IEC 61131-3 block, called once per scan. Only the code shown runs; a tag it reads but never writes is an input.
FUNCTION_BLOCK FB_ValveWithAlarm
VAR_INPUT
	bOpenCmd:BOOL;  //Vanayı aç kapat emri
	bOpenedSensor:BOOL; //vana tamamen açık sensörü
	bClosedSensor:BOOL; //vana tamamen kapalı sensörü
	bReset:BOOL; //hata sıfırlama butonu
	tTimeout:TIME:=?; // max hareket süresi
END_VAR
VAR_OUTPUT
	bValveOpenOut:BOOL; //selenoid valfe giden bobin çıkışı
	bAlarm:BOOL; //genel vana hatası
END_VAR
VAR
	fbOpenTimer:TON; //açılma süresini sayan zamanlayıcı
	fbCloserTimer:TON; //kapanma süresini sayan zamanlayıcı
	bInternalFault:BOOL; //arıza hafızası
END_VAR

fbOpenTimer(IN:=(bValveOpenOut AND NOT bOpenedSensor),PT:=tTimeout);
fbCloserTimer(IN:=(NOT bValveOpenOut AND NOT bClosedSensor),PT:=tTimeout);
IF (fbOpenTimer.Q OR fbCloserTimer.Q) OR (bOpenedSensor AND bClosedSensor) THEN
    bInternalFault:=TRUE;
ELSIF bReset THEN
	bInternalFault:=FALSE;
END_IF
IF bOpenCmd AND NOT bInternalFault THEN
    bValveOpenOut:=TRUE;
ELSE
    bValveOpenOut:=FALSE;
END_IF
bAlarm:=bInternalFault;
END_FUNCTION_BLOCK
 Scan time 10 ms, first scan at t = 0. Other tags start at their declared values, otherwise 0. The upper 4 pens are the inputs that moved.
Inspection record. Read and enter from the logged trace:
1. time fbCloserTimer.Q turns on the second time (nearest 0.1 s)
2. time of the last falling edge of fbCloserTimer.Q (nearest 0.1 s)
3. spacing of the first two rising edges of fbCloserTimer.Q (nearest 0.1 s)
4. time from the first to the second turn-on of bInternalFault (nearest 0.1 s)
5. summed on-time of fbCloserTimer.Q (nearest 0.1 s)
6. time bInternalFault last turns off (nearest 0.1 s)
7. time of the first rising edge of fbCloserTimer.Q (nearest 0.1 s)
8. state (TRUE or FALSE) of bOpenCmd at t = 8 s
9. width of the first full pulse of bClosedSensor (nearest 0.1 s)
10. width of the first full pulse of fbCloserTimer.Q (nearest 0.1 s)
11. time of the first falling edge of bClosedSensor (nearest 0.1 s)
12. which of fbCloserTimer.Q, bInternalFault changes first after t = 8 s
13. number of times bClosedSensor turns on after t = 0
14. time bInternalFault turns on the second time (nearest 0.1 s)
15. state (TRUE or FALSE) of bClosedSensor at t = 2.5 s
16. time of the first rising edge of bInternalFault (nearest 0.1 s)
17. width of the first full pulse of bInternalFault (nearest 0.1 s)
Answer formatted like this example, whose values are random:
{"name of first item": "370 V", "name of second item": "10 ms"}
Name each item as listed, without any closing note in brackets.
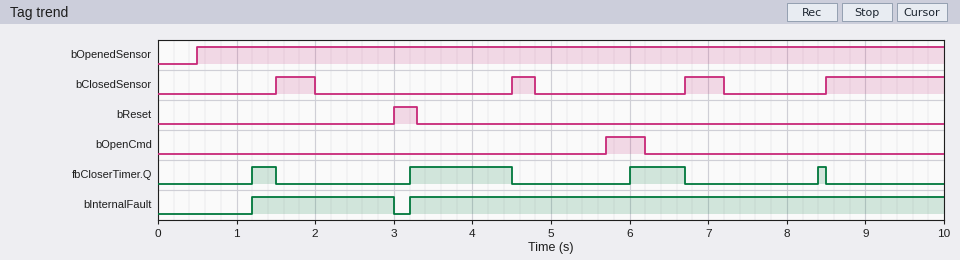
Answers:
{"time fbCloserTimer.Q turns on the second time": "3.2 s", "time of the last falling edge of fbCloserTimer.Q": "8.5 s", "spacing of the first two rising edges of fbCloserTimer.Q": "2.0 s", "time from the first to the second turn-on of bInternalFault": "2.0 s", "summed on-time of fbCloserTimer.Q": "2.4 s", "time bInternalFault last turns off": "3.0 s", "time of the first rising edge of fbCloserTimer.Q": "1.2 s", "state (TRUE or FALSE) of bOpenCmd at t = 8 s": "FALSE", "width of the first full pulse of bClosedSensor": "0.5 s", "width of the first full pulse of fbCloserTimer.Q": "0.3 s", "time of the first falling edge of bClosedSensor": "2.0 s", "which of fbCloserTimer.Q, bInternalFault changes first after t = 8 s": "fbCloserTimer.Q", "number of times bClosedSensor turns on after t = 0": "4", "time bInternalFault turns on the second time": "3.2 s", "state (TRUE or FALSE) of bClosedSensor at t = 2.5 s": "FALSE", "time of the first rising edge of bInternalFault": "1.2 s", "width of the first full pulse of bInternalFault": "1.8 s"}
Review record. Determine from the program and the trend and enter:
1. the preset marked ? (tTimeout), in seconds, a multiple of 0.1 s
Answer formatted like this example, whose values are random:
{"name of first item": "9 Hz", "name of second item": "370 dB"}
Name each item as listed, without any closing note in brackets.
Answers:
{"the preset marked ? (tTimeout), in seconds, a multiple of 0.1 s": "1.2 s"}
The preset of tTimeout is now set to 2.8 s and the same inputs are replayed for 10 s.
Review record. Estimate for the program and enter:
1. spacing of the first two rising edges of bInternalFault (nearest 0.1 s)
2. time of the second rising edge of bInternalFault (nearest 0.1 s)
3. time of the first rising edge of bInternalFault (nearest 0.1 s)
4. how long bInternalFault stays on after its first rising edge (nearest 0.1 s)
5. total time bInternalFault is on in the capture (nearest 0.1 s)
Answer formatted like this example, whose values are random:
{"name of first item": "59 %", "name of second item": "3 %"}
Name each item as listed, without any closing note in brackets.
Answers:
{"spacing of the first two rising edges of bInternalFault": "3.0 s", "time of the second rising edge of bInternalFault": "4.5 s", "time of the first rising edge of bInternalFault": "1.5 s", "how long bInternalFault stays on after its first rising edge": "1.5 s", "total time bInternalFault is on in the capture": "7.0 s"}
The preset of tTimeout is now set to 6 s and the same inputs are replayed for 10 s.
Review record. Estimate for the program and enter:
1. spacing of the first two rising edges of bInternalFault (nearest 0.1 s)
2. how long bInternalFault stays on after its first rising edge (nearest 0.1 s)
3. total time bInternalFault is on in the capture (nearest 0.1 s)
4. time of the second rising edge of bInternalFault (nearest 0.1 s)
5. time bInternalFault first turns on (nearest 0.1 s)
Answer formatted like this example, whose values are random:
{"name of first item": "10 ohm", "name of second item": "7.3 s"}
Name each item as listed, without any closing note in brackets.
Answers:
{"spacing of the first two rising edges of bInternalFault": "3.0 s", "how long bInternalFault stays on after its first rising edge": "1.5 s", "total time bInternalFault is on in the capture": "7.0 s", "time of the second rising edge of bInternalFault": "4.5 s", "time bInternalFault first turns on": "1.5 s"}
